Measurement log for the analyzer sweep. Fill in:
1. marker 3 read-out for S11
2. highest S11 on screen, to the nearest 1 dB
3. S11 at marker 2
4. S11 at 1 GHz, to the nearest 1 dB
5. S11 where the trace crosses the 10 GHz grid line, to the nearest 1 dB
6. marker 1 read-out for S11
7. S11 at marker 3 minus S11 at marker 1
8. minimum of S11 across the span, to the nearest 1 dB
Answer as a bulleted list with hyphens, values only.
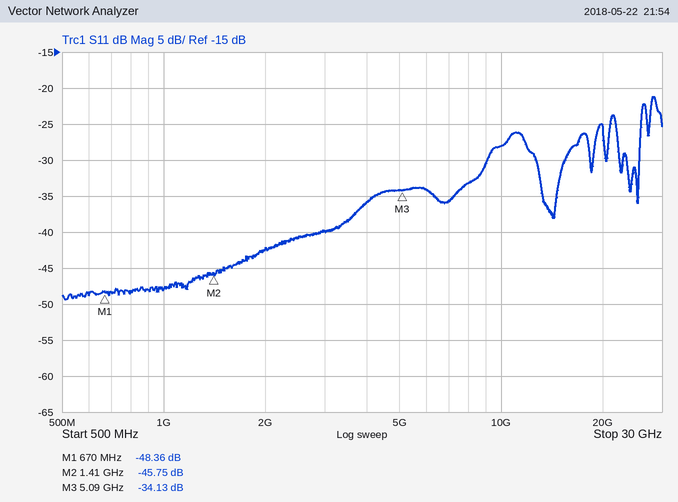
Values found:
- -34.13 dB
- -21 dB
- -45.75 dB
- -48 dB
- -28 dB
- -48.36 dB
- 14.23 dB
- -49 dB
